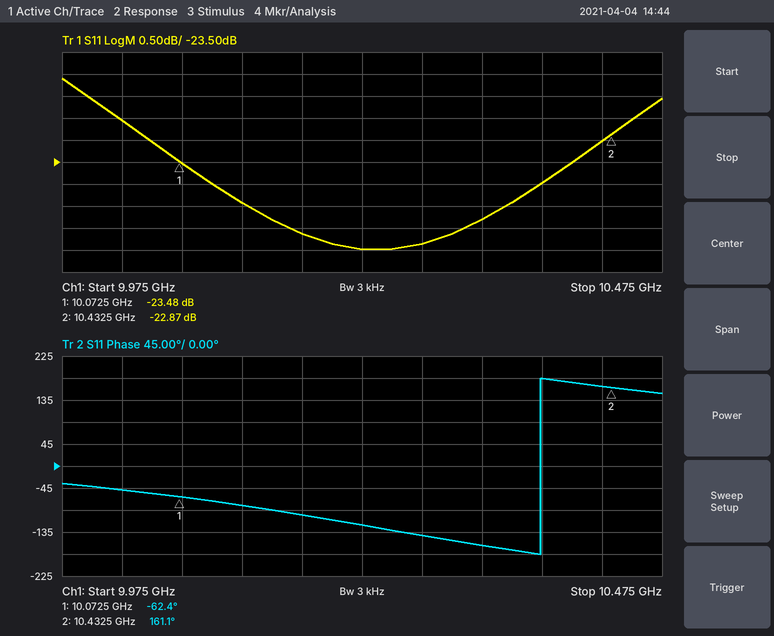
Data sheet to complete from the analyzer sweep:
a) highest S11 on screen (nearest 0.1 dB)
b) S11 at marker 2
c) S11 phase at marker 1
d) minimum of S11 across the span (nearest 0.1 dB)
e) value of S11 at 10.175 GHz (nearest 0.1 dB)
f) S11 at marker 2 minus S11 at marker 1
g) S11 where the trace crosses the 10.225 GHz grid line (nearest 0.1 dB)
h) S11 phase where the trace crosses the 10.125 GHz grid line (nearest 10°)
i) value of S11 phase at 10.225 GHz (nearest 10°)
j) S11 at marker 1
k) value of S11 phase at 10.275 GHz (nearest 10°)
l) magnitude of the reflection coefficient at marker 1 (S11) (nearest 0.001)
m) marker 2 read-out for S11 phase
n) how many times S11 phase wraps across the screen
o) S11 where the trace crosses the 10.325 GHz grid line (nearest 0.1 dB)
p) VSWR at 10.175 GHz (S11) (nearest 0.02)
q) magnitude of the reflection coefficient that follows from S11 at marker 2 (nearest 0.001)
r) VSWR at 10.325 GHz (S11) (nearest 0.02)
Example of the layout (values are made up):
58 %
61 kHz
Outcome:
-21.6 dB
-22.87 dB
-62.4°
-25.5 dB
-25.1 dB
0.61 dB
-25.5 dB
-80°
-120°
-23.48 dB
-140°
0.067
161.1°
1
-24.8 dB
1.12
0.072
1.12
